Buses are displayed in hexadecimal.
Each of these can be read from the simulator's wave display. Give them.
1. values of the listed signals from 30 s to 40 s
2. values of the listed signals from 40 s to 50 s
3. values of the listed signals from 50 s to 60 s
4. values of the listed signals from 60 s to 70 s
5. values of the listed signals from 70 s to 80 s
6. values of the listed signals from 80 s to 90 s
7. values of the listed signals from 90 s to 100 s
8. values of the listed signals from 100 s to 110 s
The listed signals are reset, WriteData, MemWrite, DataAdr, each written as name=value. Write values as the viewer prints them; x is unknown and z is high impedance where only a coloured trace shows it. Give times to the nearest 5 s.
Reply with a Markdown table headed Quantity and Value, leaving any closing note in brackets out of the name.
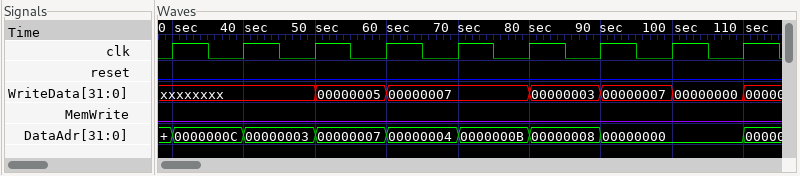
| Quantity | Value |
|---|---|
| values of the listed signals from 30 s to 40 s | reset=0, WriteData=xxxxxxxx, MemWrite=0, DataAdr=0000000C |
| values of the listed signals from 40 s to 50 s | reset=0, WriteData=xxxxxxxx, MemWrite=0, DataAdr=00000003 |
| values of the listed signals from 50 s to 60 s | reset=0, WriteData=00000005, MemWrite=0, DataAdr=00000007 |
| values of the listed signals from 60 s to 70 s | reset=0, WriteData=00000007, MemWrite=0, DataAdr=00000004 |
| values of the listed signals from 70 s to 80 s | reset=0, WriteData=00000007, MemWrite=0, DataAdr=0000000B |
| values of the listed signals from 80 s to 90 s | reset=0, WriteData=00000003, MemWrite=0, DataAdr=00000008 |
| values of the listed signals from 90 s to 100 s | reset=0, WriteData=00000007, MemWrite=0, DataAdr=00000000 |
| values of the listed signals from 100 s to 110 s | reset=0, WriteData=00000000, MemWrite=0, DataAdr=00000000 |
